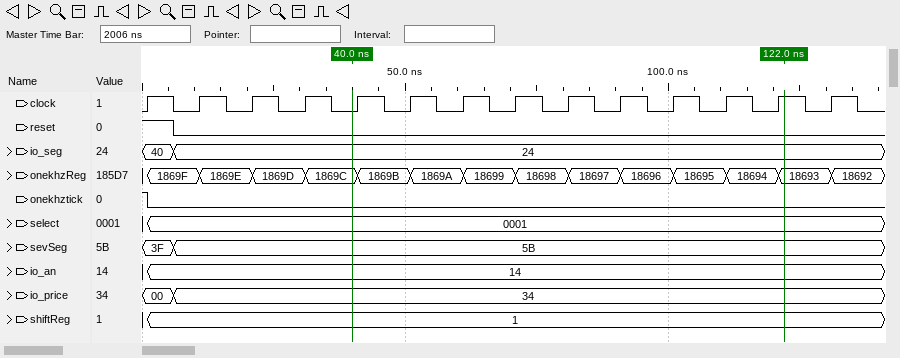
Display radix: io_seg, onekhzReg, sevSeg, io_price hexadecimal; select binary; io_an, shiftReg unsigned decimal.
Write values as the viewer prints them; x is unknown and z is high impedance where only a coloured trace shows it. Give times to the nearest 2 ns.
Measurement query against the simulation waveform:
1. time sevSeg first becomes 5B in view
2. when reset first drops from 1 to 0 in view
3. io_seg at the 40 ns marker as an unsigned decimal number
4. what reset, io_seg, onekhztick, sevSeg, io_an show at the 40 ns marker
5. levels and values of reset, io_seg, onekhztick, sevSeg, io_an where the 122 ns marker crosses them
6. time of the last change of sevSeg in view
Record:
6 ns
6 ns
36
reset=0, io_seg=24, onekhztick=0, sevSeg=5B, io_an=14
reset=0, io_seg=24, onekhztick=0, sevSeg=5B, io_an=14
6 ns
